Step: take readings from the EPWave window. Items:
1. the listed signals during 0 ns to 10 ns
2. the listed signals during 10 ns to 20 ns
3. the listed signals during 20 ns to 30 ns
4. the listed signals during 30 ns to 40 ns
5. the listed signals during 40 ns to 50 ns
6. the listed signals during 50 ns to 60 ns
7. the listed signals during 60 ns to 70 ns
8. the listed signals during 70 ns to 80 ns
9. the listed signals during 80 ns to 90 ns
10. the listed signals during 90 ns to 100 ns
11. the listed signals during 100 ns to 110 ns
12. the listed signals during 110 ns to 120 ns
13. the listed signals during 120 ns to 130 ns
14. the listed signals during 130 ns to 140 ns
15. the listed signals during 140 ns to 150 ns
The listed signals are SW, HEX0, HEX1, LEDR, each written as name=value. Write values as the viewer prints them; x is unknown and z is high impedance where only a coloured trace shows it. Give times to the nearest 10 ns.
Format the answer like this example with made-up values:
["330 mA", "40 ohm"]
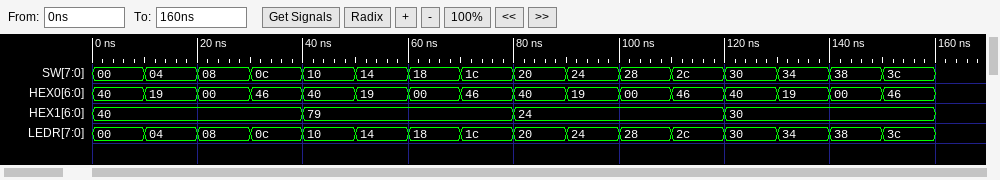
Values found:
["SW=00, HEX0=40, HEX1=40, LEDR=00", "SW=04, HEX0=19, HEX1=40, LEDR=04", "SW=08, HEX0=00, HEX1=40, LEDR=08", "SW=0c, HEX0=46, HEX1=40, LEDR=0c", "SW=10, HEX0=40, HEX1=79, LEDR=10", "SW=14, HEX0=19, HEX1=79, LEDR=14", "SW=18, HEX0=00, HEX1=79, LEDR=18", "SW=1c, HEX0=46, HEX1=79, LEDR=1c", "SW=20, HEX0=40, HEX1=24, LEDR=20", "SW=24, HEX0=19, HEX1=24, LEDR=24", "SW=28, HEX0=00, HEX1=24, LEDR=28", "SW=2c, HEX0=46, HEX1=24, LEDR=2c", "SW=30, HEX0=40, HEX1=30, LEDR=30", "SW=34, HEX0=19, HEX1=30, LEDR=34", "SW=38, HEX0=00, HEX1=30, LEDR=38"]
